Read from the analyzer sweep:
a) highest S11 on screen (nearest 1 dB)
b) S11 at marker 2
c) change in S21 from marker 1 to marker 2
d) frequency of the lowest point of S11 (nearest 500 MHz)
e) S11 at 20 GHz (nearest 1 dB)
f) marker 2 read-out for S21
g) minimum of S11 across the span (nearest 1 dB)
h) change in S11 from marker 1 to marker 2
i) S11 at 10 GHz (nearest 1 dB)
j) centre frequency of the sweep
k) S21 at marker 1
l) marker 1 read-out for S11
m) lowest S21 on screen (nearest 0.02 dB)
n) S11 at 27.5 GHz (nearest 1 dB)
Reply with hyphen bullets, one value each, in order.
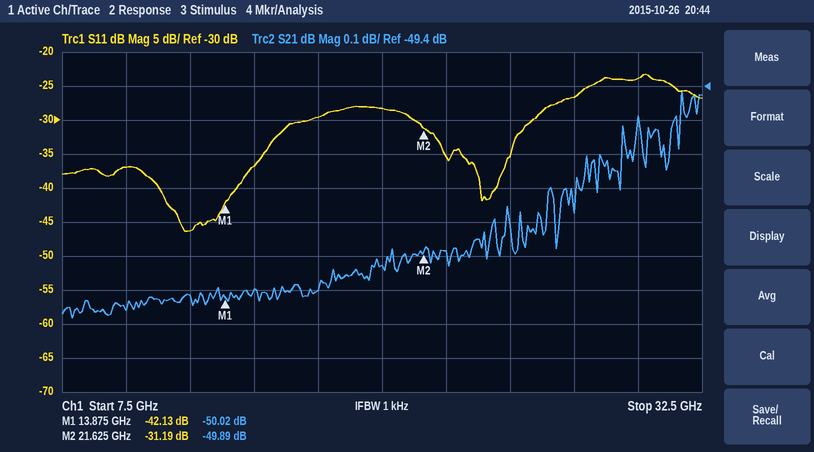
- -23 dB
- -31.19 dB
- 0.13 dB
- 12.5 GHz
- -28 dB
- -49.89 dB
- -46 dB
- 10.94 dB
- -37 dB
- 20 GHz
- -50.02 dB
- -42.13 dB
- -50.08 dB
- -27 dB
